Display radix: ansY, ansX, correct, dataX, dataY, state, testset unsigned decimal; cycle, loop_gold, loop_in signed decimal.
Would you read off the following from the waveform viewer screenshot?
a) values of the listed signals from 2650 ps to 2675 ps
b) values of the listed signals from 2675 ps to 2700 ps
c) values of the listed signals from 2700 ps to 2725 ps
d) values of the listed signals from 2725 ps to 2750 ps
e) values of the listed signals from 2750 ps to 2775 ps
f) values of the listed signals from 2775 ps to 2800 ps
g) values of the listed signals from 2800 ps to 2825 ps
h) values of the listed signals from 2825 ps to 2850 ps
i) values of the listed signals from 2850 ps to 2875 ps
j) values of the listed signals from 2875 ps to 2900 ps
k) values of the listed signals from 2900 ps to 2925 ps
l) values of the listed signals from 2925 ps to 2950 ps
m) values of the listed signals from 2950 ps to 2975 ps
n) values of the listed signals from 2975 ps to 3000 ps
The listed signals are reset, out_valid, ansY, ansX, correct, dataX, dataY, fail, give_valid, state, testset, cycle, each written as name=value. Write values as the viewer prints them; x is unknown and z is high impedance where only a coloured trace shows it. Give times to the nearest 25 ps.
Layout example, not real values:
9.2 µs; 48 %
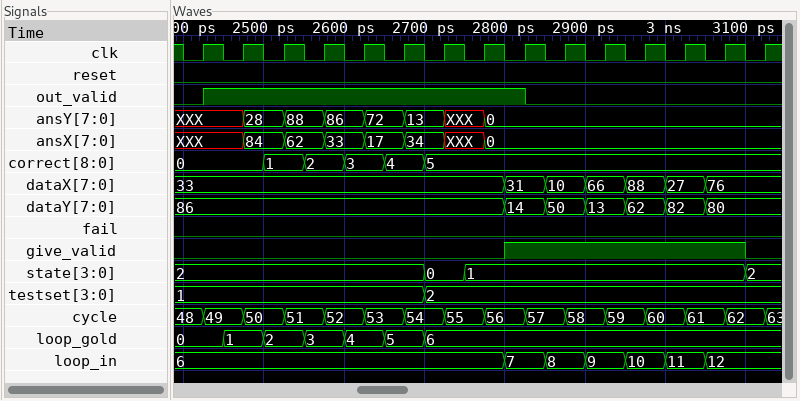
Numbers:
reset=0, out_valid=1, ansY=72, ansX=17, correct=4, dataX=33, dataY=86, fail=0, give_valid=0, state=2, testset=1, cycle=53; reset=0, out_valid=1, ansY=13, ansX=34, correct=4, dataX=33, dataY=86, fail=0, give_valid=0, state=2, testset=1, cycle=54; reset=0, out_valid=1, ansY=13, ansX=34, correct=5, dataX=33, dataY=86, fail=0, give_valid=0, state=0, testset=2, cycle=54; reset=0, out_valid=1, ansY=XXX, ansX=XXX, correct=5, dataX=33, dataY=86, fail=0, give_valid=0, state=0, testset=2, cycle=55; reset=0, out_valid=1, ansY=XXX, ansX=XXX, correct=5, dataX=33, dataY=86, fail=0, give_valid=0, state=1, testset=2, cycle=55; reset=0, out_valid=1, ansY=0, ansX=0, correct=5, dataX=33, dataY=86, fail=0, give_valid=0, state=1, testset=2, cycle=56; reset=0, out_valid=1, ansY=0, ansX=0, correct=5, dataX=31, dataY=14, fail=0, give_valid=1, state=1, testset=2, cycle=56; reset=0, out_valid=0, ansY=0, ansX=0, correct=5, dataX=31, dataY=14, fail=0, give_valid=1, state=1, testset=2, cycle=57; reset=0, out_valid=0, ansY=0, ansX=0, correct=5, dataX=10, dataY=50, fail=0, give_valid=1, state=1, testset=2, cycle=57; reset=0, out_valid=0, ansY=0, ansX=0, correct=5, dataX=10, dataY=50, fail=0, give_valid=1, state=1, testset=2, cycle=58; reset=0, out_valid=0, ansY=0, ansX=0, correct=5, dataX=66, dataY=13, fail=0, give_valid=1, state=1, testset=2, cycle=58; reset=0, out_valid=0, ansY=0, ansX=0, correct=5, dataX=66, dataY=13, fail=0, give_valid=1, state=1, testset=2, cycle=59; reset=0, out_valid=0, ansY=0, ansX=0, correct=5, dataX=88, dataY=62, fail=0, give_valid=1, state=1, testset=2, cycle=59; reset=0, out_valid=0, ansY=0, ansX=0, correct=5, dataX=88, dataY=62, fail=0, give_valid=1, state=1, testset=2, cycle=60
